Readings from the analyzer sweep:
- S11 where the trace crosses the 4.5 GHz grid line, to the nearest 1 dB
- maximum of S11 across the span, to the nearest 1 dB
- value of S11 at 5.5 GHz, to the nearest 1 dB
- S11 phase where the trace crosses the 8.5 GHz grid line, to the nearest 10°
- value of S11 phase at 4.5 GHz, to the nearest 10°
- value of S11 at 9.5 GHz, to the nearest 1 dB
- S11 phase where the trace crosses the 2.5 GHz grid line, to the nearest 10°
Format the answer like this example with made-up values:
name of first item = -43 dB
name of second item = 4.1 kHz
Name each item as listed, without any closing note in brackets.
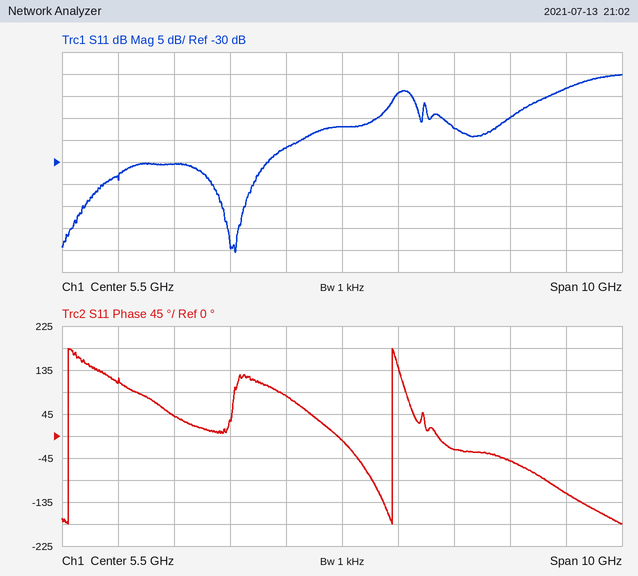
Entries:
S11 where the trace crosses the 4.5 GHz grid line, to the nearest 1 dB = -27 dB
maximum of S11 across the span, to the nearest 1 dB = -10 dB
value of S11 at 5.5 GHz, to the nearest 1 dB = -22 dB
S11 phase where the trace crosses the 8.5 GHz grid line, to the nearest 10° = -50°
value of S11 phase at 4.5 GHz, to the nearest 10° = 80°
value of S11 at 9.5 GHz, to the nearest 1 dB = -13 dB
S11 phase where the trace crosses the 2.5 GHz grid line, to the nearest 10° = 40°
